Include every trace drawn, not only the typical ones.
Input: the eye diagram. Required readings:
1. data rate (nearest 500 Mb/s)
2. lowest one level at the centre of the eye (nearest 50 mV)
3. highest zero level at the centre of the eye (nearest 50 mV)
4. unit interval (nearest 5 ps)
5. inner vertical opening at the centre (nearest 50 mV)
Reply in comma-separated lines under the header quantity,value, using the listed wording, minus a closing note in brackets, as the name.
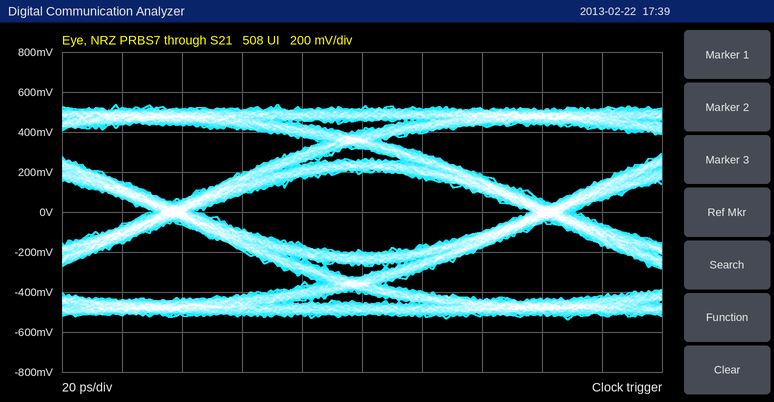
quantity,value
data rate,8.0 Gb/s
lowest one level at the centre of the eye,200 mV
highest zero level at the centre of the eye,-200 mV
unit interval,125 ps
inner vertical opening at the centre,400 mV
